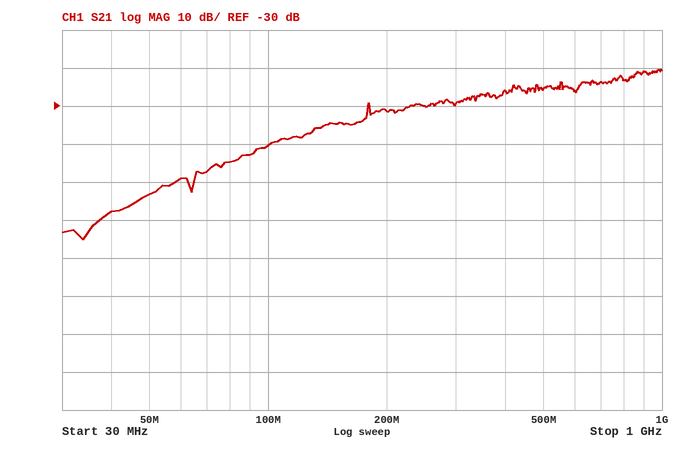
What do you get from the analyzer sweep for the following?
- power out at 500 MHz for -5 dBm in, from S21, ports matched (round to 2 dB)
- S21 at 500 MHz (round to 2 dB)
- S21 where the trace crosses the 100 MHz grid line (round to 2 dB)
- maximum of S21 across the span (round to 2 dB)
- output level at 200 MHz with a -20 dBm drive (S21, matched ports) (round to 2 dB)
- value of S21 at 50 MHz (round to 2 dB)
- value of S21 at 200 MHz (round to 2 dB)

-30 dBm
-26 dB
-40 dB
-20 dB
-52 dBm
-54 dB
-32 dB
